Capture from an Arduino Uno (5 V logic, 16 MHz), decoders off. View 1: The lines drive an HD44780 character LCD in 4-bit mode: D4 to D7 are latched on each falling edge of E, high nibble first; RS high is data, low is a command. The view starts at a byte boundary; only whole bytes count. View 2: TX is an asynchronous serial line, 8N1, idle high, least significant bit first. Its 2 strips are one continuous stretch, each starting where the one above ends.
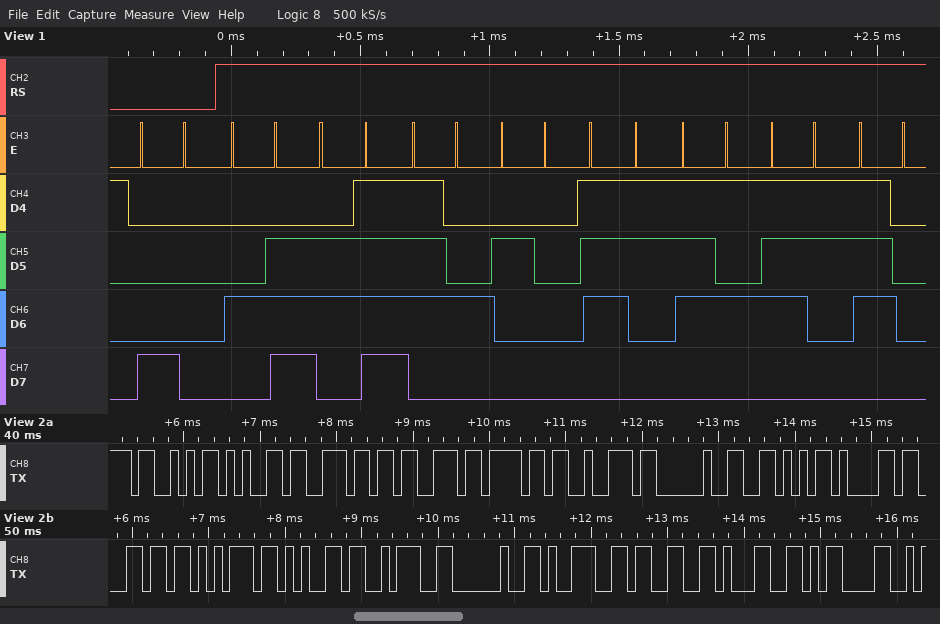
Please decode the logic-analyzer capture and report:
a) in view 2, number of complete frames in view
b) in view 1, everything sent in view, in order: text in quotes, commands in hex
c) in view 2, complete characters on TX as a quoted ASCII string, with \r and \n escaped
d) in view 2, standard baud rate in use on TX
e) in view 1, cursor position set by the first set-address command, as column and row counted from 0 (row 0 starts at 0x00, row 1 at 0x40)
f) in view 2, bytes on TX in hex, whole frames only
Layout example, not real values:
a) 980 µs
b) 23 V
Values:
a) 18
b) 0x80 "Not susp"
c) "Sensor Value: 931\r"
d) 9600 baud
e) column 0, row 0
f) 53 65 6E 73 6F 72 20 56 61 6C 75 65 3A 20 39 33 31 0D
